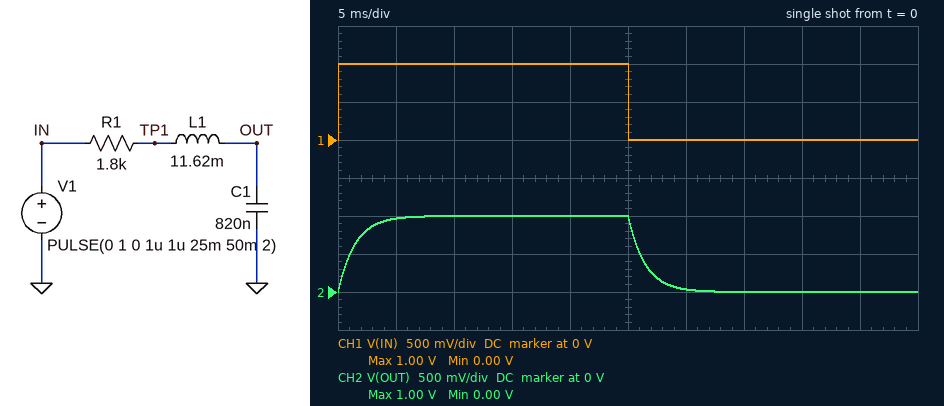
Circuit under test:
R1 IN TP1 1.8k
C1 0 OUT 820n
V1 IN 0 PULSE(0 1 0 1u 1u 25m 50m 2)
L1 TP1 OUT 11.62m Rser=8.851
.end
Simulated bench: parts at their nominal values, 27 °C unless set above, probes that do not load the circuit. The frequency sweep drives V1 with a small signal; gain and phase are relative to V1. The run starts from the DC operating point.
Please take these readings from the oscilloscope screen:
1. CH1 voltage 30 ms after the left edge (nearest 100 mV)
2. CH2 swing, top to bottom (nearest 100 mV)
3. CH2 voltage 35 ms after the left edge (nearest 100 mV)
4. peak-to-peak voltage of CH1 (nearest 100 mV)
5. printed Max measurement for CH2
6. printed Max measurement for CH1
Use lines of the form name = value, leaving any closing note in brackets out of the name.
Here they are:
CH1 voltage 30 ms after the left edge = 0 V
CH2 swing, top to bottom = 1.0 V
CH2 voltage 35 ms after the left edge = 0 V
peak-to-peak voltage of CH1 = 1.0 V
printed Max measurement for CH2 = 1.00 V
printed Max measurement for CH1 = 1.00 V
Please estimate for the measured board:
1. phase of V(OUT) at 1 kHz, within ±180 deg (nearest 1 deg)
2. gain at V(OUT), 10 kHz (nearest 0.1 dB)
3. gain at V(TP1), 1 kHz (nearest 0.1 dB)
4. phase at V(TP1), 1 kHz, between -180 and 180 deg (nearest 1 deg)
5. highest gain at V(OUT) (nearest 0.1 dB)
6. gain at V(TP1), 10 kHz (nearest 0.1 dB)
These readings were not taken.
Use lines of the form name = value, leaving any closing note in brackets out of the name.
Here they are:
phase of V(OUT) at 1 kHz, within ±180 deg = -86 deg
gain at V(OUT), 10 kHz = -40.0 dB
gain at V(TP1), 1 kHz = -23.5 dB
phase at V(TP1), 1 kHz, between -180 and 180 deg = -82 deg
highest gain at V(OUT) = 0 dB
gain at V(TP1), 10 kHz = -8.7 dB
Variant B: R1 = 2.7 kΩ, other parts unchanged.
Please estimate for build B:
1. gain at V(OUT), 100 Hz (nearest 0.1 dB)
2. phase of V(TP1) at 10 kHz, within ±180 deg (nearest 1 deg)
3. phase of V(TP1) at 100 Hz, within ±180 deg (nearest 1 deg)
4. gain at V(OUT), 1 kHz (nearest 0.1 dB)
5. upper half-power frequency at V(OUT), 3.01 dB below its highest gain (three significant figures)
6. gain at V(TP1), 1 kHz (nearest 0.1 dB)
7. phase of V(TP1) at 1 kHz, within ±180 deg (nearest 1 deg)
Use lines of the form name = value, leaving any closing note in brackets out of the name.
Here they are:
gain at V(OUT), 100 Hz = -4.7 dB
phase of V(TP1) at 10 kHz, within ±180 deg = 75 deg
phase of V(TP1) at 100 Hz, within ±180 deg = -54 deg
gain at V(OUT), 1 kHz = -22.9 dB
upper half-power frequency at V(OUT), 3.01 dB below its highest gain = 71.8 Hz
gain at V(TP1), 1 kHz = -27.0 dB
phase of V(TP1) at 1 kHz, within ±180 deg = -83 deg
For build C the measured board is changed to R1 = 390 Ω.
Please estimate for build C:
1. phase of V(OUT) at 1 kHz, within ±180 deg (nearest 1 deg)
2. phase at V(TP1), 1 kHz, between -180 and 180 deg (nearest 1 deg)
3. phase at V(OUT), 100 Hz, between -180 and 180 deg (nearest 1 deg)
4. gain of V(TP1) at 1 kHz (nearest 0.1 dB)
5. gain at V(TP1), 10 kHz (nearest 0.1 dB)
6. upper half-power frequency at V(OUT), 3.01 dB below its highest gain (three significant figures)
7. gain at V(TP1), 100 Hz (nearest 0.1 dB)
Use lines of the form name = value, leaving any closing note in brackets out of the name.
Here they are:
phase of V(OUT) at 1 kHz, within ±180 deg = -73 deg
phase at V(TP1), 1 kHz, between -180 and 180 deg = -69 deg
phase at V(OUT), 100 Hz, between -180 and 180 deg = -12 deg
gain of V(TP1) at 1 kHz = -10.7 dB
gain at V(TP1), 10 kHz = -1.2 dB
upper half-power frequency at V(OUT), 3.01 dB below its highest gain = 534 Hz
gain at V(TP1), 100 Hz = -0.2 dB
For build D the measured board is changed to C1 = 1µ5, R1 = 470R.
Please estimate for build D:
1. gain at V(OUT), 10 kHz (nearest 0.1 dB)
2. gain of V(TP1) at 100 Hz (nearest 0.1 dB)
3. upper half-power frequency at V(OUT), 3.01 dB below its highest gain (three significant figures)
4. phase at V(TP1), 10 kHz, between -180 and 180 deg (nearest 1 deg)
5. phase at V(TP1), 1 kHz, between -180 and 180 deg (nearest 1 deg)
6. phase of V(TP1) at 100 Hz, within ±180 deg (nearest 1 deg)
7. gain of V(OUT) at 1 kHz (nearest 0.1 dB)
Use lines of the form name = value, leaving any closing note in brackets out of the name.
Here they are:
gain at V(OUT), 10 kHz = -38.2 dB
gain of V(TP1) at 100 Hz = -0.8 dB
upper half-power frequency at V(OUT), 3.01 dB below its highest gain = 229 Hz
phase at V(TP1), 10 kHz, between -180 and 180 deg = 33 deg
phase at V(TP1), 1 kHz, between -180 and 180 deg = -71 deg
phase of V(TP1) at 100 Hz, within ±180 deg = -24 deg
gain of V(OUT) at 1 kHz = -13.1 dB
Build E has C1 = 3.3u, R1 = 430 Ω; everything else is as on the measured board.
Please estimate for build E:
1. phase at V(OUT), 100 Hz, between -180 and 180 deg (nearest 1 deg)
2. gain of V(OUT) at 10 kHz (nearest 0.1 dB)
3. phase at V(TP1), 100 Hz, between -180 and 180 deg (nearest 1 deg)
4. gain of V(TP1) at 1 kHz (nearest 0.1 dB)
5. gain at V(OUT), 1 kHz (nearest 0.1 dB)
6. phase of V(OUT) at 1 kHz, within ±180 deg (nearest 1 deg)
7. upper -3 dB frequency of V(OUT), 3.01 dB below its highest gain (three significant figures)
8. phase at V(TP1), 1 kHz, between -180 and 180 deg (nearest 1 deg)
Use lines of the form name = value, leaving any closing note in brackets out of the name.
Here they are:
phase at V(OUT), 100 Hz, between -180 and 180 deg = -43 deg
gain of V(OUT) at 10 kHz = -44.9 dB
phase at V(TP1), 100 Hz, between -180 and 180 deg = -42 deg
gain of V(TP1) at 1 kHz = -24.5 dB
gain at V(OUT), 1 kHz = -19.2 dB
phase of V(OUT) at 1 kHz, within ±180 deg = -93 deg
upper -3 dB frequency of V(OUT), 3.01 dB below its highest gain = 112 Hz
phase at V(TP1), 1 kHz, between -180 and 180 deg = 67 deg
